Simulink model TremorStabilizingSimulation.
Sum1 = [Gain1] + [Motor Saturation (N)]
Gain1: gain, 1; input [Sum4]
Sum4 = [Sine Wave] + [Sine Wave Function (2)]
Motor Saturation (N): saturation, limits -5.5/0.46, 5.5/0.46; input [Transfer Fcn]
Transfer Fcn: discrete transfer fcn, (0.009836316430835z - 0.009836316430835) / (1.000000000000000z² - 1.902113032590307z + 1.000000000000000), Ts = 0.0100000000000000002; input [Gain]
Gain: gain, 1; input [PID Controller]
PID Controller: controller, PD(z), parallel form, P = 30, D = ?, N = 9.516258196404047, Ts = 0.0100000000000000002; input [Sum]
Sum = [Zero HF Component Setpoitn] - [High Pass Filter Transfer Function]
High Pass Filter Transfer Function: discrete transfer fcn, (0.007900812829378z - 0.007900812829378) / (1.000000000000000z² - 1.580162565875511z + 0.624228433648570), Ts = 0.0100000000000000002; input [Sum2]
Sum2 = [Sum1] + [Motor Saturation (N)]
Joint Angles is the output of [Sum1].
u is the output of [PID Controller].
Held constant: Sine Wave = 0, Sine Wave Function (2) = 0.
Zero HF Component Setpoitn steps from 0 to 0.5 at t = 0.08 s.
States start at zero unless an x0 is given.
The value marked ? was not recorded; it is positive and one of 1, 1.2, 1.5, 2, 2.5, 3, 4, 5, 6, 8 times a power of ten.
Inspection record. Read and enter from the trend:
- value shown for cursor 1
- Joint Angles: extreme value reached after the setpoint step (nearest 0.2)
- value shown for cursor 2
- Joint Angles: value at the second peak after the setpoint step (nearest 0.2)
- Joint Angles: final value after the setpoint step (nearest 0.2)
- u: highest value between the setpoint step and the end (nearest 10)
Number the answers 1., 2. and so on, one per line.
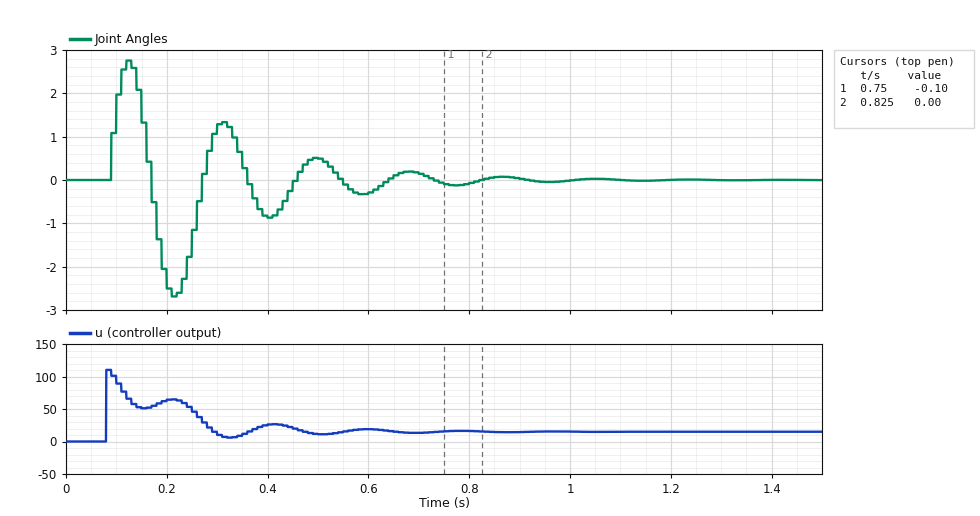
1. -0.10
2. 2.8
3. 0.00
4. 1.4
5. 0.0
6. 110
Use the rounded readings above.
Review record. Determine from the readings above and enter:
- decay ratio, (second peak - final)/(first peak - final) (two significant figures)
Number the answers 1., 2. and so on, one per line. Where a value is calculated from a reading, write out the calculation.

1. (1.4 - 0) / (2.8 - 0) = 0.50
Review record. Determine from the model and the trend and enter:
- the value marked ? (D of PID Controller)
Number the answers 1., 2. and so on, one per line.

1. 20
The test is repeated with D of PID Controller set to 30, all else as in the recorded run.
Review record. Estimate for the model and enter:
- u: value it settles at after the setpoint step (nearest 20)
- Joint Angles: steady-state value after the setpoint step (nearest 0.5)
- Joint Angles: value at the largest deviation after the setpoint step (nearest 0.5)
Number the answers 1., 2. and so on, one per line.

1. 20
2. 0.0
3. 4.0
